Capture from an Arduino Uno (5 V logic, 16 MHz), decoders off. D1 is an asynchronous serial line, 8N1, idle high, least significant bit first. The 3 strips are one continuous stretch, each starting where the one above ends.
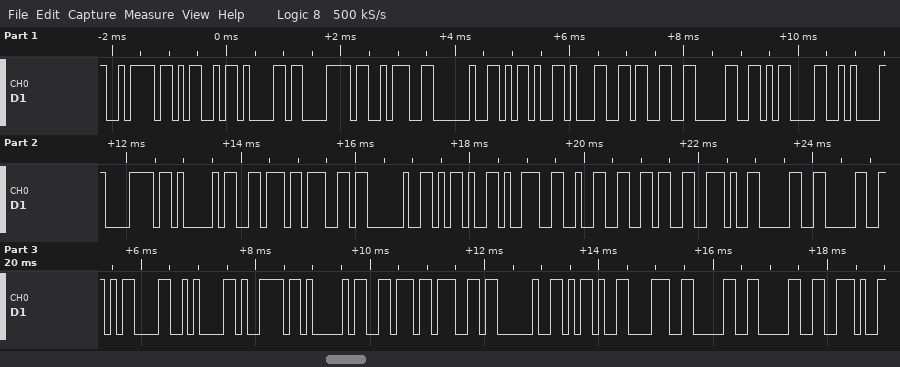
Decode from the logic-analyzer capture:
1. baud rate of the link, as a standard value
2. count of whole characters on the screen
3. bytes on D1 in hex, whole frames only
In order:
9600 baud
36
7A 4D 61 78 3A 20 2D 31 33 30 0D 0A 78 41 76 67 20 2D 39 32 36 2E 30 30 0D 0A 79 41 76 67 20 2D 38 30 30 2E
